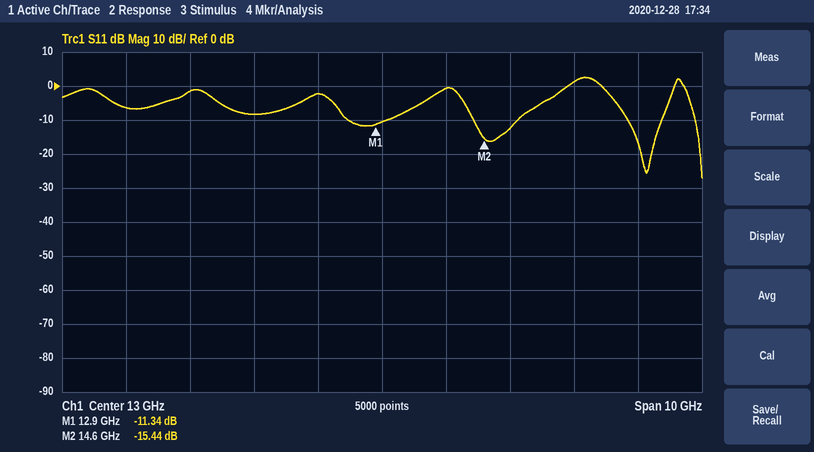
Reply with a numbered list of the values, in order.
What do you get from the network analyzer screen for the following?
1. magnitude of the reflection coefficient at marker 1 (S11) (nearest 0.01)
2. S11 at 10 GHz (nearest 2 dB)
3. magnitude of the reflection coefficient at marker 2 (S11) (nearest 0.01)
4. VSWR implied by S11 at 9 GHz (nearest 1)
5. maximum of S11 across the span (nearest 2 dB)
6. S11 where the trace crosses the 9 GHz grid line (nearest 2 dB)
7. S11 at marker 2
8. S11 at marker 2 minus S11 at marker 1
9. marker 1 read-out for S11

1. 0.27
2. -2 dB
3. 0.17
4. 3
5. 2 dB
6. -6 dB
7. -15.44 dB
8. -4.10 dB
9. -11.34 dB
